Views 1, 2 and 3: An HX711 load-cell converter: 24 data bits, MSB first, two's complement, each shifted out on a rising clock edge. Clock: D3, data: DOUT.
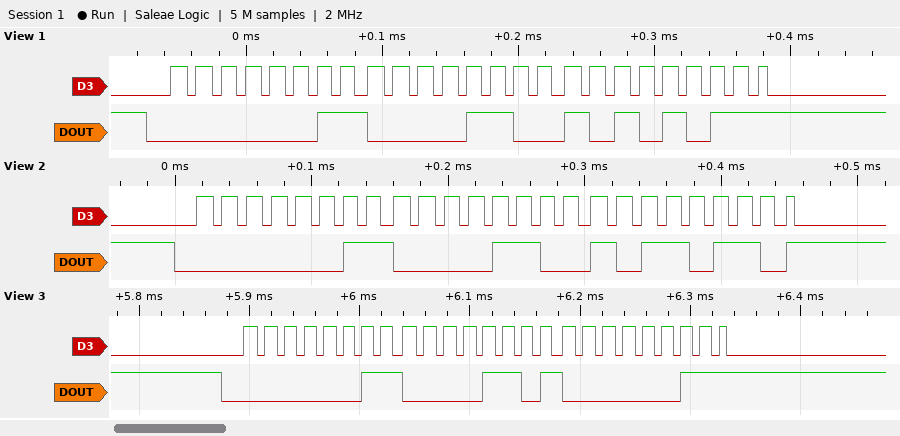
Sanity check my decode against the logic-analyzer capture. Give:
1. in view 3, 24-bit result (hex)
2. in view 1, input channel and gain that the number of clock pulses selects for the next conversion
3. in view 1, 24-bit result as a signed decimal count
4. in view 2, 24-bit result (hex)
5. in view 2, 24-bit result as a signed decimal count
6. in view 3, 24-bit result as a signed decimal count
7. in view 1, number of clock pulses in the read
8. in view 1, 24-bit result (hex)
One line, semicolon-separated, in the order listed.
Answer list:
0x030D03; channel A, gain 128; 199851; 0x030CB6; 199862; 199939; 25; 0x030CAB
